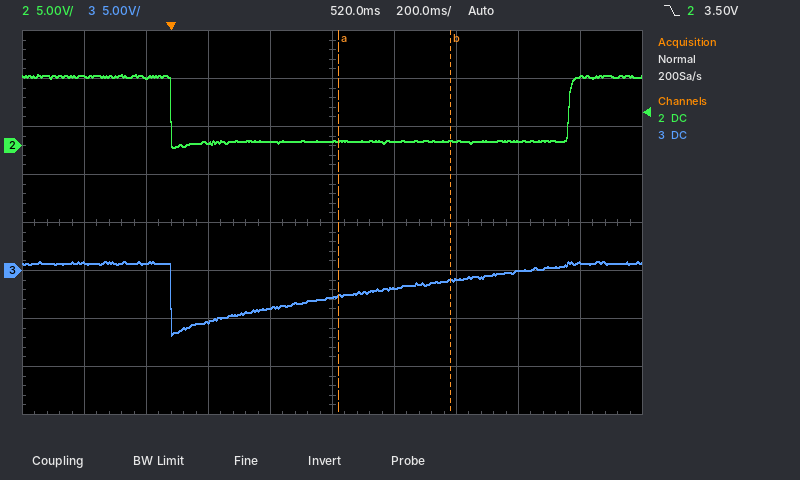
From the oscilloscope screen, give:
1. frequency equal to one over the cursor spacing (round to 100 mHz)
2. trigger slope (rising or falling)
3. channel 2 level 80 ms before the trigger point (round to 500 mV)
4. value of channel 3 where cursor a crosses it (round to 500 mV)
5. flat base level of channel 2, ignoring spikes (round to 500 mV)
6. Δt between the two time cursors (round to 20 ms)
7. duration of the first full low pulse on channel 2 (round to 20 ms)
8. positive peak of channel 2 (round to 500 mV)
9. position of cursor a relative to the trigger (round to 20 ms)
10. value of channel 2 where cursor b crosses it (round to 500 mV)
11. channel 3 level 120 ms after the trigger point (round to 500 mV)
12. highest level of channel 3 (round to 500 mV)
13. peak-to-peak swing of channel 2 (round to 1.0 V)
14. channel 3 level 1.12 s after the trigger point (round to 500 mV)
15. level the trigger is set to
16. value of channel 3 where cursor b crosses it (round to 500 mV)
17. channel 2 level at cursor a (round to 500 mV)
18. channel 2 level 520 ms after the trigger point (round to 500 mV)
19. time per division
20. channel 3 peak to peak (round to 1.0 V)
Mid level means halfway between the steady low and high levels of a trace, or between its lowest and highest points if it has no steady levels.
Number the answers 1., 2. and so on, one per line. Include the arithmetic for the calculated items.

1. 1 / 360 ms ≈ 2.8 Hz
2. falling
3. 7.0 V
4. -2.5 V
5. 500 mV
6. 360 ms
7. 1.28 s
8. 7.5 V
9. +540 ms
10. 500 mV
11. -5.5 V
12. 1.0 V
13. 8.0 V
14. 0.0 V
15. 3.50 V
16. -1.0 V
17. 500 mV
18. 500 mV
19. 200 ms
20. 8.0 V
